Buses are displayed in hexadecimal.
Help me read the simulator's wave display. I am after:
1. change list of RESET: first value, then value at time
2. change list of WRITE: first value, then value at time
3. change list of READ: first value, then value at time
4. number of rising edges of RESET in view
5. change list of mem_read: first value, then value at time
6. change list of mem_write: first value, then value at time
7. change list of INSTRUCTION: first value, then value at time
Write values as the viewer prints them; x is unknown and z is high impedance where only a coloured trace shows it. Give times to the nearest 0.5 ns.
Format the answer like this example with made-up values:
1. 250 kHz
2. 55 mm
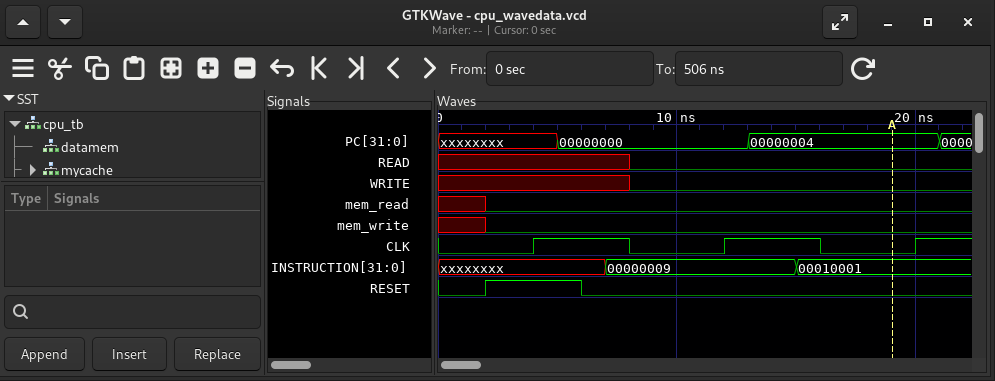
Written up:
1. 0, 1 at 2 ns, 0 at 6 ns
2. x, 0 at 8 ns
3. x, 0 at 8 ns
4. 1
5. x, 0 at 2 ns
6. x, 0 at 2 ns
7. xxxxxxxx, 00000009 at 7 ns, 00010001 at 15 ns
